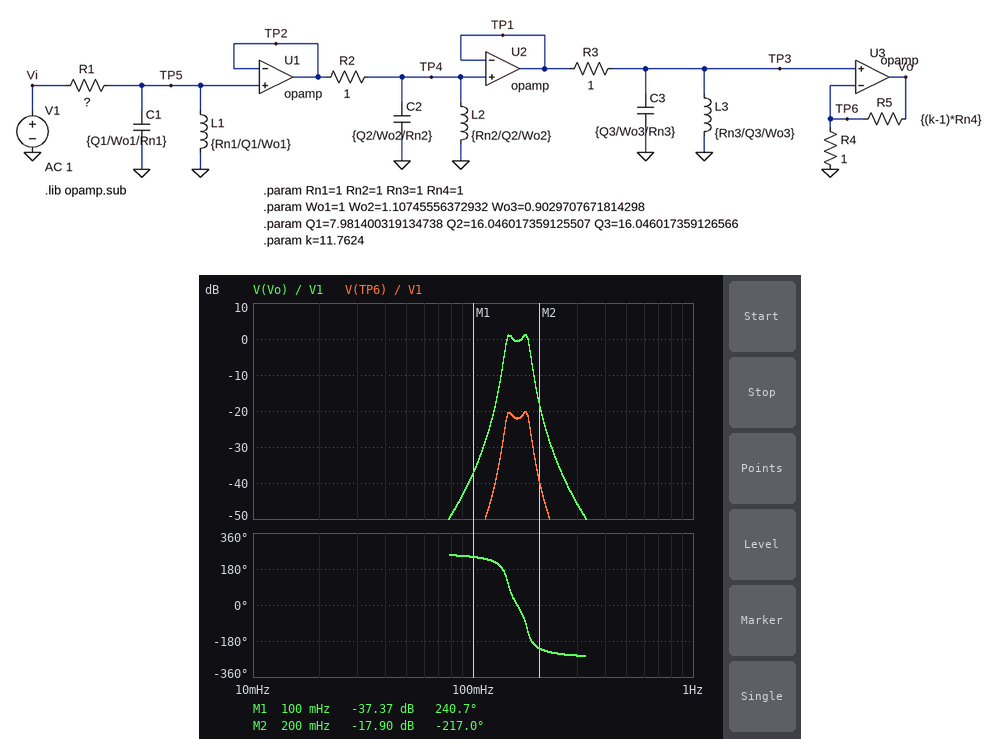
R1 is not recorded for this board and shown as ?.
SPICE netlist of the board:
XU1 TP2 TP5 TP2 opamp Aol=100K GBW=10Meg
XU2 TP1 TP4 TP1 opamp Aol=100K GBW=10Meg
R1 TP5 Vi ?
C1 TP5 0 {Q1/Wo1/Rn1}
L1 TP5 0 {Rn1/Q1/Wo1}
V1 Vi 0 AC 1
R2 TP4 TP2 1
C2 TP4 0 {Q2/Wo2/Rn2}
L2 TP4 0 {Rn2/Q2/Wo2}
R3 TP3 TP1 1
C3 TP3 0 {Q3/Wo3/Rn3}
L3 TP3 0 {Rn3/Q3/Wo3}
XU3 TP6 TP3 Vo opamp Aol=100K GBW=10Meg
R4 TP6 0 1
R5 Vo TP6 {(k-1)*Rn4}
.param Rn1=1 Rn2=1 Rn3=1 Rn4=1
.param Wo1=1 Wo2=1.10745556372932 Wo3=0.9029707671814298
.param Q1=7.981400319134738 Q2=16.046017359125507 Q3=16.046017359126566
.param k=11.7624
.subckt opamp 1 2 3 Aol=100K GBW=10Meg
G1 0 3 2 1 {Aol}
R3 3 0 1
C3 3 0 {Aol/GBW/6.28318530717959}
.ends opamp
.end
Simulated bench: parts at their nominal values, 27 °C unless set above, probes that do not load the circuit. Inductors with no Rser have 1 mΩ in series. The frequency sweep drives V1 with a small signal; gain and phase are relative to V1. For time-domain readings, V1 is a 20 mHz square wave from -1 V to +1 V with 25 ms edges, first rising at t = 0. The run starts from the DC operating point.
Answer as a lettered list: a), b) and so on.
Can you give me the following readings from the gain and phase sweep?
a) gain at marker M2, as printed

a) -17.90 dB
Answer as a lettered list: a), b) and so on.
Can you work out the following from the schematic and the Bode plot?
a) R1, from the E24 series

a) 0.47 Ω
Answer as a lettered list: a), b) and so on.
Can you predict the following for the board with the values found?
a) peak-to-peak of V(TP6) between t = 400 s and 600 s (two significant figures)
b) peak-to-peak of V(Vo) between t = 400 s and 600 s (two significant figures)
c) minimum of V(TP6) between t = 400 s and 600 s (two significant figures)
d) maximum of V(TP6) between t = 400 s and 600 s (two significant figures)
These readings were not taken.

a) 40 mV
b) 470 mV
c) -20 mV
d) 20 mV
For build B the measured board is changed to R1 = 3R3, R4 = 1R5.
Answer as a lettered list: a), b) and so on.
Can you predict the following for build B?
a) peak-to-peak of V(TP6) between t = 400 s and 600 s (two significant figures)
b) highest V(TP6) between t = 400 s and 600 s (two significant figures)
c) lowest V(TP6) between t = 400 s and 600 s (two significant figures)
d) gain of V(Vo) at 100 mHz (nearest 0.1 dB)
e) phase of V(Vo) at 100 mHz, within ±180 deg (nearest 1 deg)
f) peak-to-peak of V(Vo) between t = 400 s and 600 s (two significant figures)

a) 8.8 mV
b) 4.4 mV
c) -4.4 mV
d) -57.1 dB
e) -106 deg
f) 72 mV
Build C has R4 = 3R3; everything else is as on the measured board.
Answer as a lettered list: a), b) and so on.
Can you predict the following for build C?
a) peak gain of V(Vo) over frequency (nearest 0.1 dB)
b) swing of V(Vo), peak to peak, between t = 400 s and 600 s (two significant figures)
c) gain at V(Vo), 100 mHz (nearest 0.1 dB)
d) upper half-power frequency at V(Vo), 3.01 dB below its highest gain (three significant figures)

a) -7.6 dB
b) 170 mV
c) -46.2 dB
d) 180 mHz
